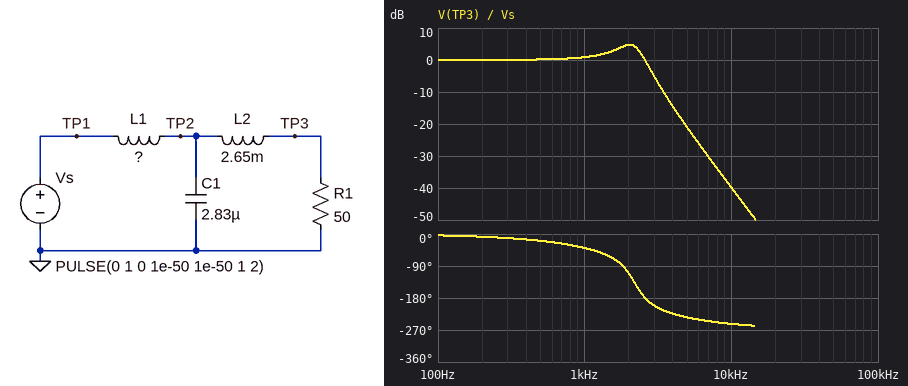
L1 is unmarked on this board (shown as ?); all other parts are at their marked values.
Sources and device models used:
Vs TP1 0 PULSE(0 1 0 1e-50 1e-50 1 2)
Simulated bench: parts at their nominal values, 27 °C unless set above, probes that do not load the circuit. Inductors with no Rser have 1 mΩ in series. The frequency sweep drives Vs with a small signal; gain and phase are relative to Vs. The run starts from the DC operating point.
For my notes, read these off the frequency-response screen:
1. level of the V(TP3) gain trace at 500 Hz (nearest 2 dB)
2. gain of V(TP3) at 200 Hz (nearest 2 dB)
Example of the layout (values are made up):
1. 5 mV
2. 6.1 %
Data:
1. 0 dB
2. 0 dB
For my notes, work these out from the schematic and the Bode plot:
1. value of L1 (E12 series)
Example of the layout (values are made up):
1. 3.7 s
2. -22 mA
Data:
1. 2.7 mH
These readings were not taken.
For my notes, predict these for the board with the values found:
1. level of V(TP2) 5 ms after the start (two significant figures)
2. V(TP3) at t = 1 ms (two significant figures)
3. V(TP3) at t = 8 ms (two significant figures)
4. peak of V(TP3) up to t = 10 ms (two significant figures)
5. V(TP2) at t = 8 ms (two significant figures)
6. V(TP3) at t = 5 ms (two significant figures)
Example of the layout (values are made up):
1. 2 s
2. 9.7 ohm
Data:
1. 1.0 V
2. 960 mV
3. 1.0 V
4. 1.3 V
5. 1.0 V
6. 1.0 V
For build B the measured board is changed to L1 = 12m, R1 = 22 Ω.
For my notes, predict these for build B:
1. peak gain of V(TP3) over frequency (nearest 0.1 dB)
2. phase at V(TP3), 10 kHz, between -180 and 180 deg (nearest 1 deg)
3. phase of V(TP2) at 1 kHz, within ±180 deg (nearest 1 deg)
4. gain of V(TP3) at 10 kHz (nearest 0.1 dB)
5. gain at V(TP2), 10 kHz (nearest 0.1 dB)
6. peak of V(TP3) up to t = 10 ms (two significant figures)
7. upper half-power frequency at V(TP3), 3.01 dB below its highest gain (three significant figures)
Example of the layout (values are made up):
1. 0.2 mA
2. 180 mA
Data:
1. 0 dB
2. 98 deg
3. -59 deg
4. -59.8 dB
5. -42.2 dB
6. 1.0 V
7. 264 Hz
